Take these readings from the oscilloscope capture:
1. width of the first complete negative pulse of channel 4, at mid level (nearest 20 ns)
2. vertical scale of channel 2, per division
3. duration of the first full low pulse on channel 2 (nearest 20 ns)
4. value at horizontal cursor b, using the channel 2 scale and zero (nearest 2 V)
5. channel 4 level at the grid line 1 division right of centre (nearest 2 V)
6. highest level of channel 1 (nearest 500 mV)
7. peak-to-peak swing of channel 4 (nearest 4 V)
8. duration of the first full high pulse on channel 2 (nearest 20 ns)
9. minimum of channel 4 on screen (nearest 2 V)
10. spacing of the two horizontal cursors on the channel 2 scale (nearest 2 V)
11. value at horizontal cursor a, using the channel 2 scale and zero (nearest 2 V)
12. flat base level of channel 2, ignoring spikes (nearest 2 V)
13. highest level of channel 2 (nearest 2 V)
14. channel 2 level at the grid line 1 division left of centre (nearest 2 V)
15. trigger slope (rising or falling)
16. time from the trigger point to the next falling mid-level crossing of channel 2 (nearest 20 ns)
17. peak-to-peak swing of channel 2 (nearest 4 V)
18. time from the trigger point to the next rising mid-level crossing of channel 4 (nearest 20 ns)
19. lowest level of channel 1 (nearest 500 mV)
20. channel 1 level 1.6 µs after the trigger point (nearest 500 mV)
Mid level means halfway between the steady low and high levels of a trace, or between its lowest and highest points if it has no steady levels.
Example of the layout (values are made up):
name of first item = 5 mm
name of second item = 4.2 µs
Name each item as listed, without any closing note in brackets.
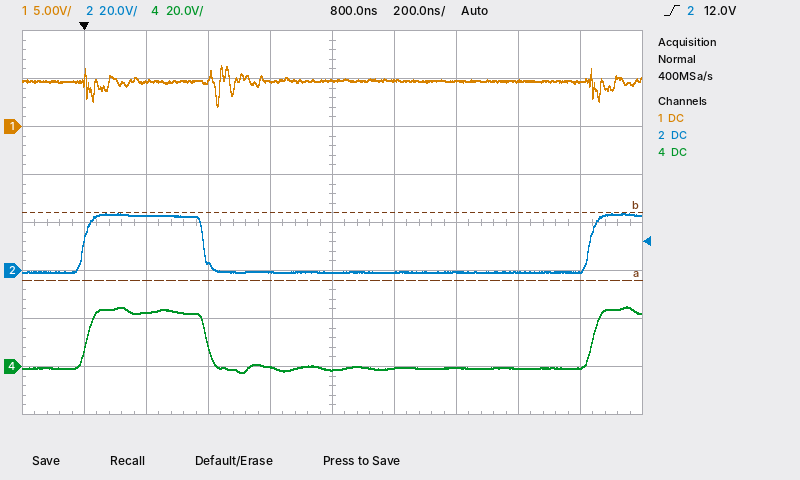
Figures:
width of the first complete negative pulse of channel 4, at mid level = 1.24 µs
vertical scale of channel 2, per division = 20 V
duration of the first full low pulse on channel 2 = 1.24 µs
value at horizontal cursor b, using the channel 2 scale and zero = 24 V
channel 4 level at the grid line 1 division right of centre = 0 V
highest level of channel 1 = 6.5 V
peak-to-peak swing of channel 4 = 28 V
duration of the first full high pulse on channel 2 = 380 ns
minimum of channel 4 on screen = -2 V
spacing of the two horizontal cursors on the channel 2 scale = 28 V
value at horizontal cursor a, using the channel 2 scale and zero = -4 V
flat base level of channel 2, ignoring spikes = 0 V
highest level of channel 2 = 24 V
channel 2 level at the grid line 1 division left of centre = 0 V
trigger slope = rising
time from the trigger point to the next falling mid-level crossing of channel 2 = 380 ns
peak-to-peak swing of channel 2 = 24 V
time from the trigger point to the next rising mid-level crossing of channel 4 = 1.64 µs
lowest level of channel 1 = 2.0 V
channel 1 level 1.6 µs after the trigger point = 4.5 V
